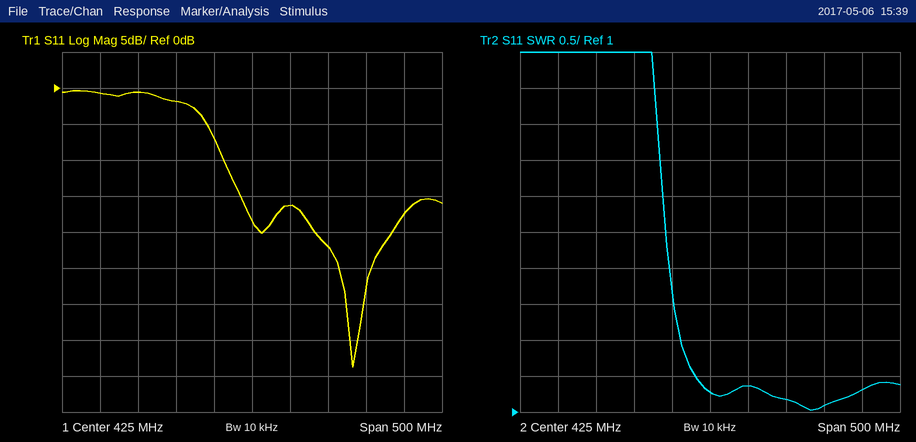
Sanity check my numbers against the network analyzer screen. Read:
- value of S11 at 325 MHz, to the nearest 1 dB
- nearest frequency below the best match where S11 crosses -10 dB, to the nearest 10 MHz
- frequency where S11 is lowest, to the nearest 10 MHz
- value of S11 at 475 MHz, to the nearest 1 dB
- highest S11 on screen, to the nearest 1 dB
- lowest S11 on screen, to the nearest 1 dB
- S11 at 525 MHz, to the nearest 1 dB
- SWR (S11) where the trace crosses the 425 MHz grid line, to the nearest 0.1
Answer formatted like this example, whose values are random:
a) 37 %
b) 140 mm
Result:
a) -2 dB
b) 390 MHz
c) 560 MHz
d) -16 dB
e) 0 dB
f) -39 dB
g) -22 dB
h) 1.3
